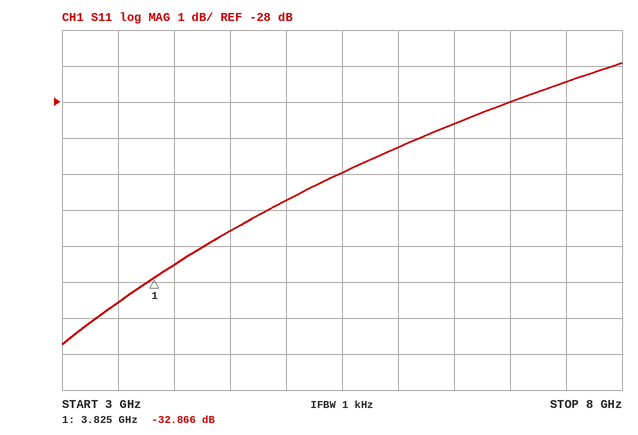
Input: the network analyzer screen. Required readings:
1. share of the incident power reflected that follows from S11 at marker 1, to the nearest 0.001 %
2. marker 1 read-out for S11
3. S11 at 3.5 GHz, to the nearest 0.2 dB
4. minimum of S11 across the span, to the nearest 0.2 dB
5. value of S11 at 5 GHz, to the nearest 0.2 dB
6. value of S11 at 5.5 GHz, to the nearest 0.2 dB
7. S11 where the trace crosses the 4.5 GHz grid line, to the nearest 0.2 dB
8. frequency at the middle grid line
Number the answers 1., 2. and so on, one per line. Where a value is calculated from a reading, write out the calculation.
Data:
1. 10^(-32.866/10) ≈ 0.052 %
2. -32.866 dB
3. -33.6 dB
4. -34.8 dB
5. -30.8 dB
6. -30.0 dB
7. -31.6 dB
8. 5.5 GHz
